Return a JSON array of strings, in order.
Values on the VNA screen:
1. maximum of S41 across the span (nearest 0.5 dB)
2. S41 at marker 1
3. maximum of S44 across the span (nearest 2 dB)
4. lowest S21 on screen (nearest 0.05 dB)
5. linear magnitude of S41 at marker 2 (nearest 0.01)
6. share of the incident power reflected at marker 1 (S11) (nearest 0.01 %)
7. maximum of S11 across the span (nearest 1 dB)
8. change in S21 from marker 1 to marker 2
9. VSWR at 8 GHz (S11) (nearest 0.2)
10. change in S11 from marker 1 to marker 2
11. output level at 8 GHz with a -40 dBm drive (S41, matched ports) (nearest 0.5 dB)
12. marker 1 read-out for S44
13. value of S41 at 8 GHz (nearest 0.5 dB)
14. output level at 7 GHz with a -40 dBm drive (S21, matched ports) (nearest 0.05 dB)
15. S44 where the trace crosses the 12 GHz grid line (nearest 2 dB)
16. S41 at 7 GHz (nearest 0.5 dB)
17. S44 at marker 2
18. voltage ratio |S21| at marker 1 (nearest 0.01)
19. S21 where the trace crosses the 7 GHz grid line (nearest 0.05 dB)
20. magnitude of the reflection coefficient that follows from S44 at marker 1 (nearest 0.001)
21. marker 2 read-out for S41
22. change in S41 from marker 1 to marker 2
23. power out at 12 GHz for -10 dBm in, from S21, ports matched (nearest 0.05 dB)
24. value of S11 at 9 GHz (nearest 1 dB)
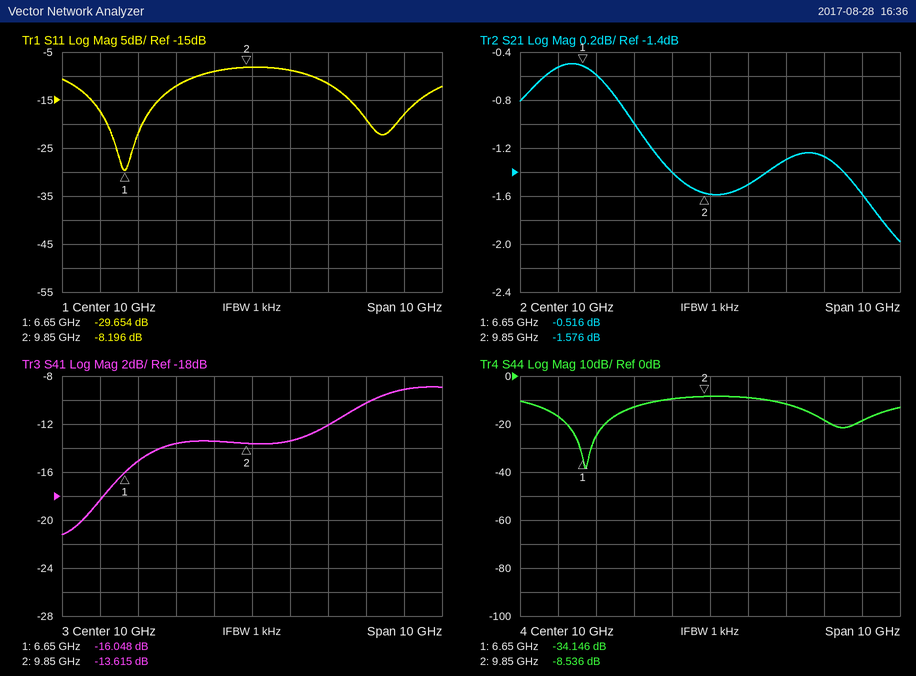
["-9.0 dB", "-16.048 dB", "-8 dB", "-2.00 dB", "0.21", "0.11 %", "-8 dB", "-1.060 dB", "1.6", "21.458 dB", "-53.5 dBm", "-34.146 dB", "-13.5 dB", "-40.60 dBm", "-12 dB", "-15.0 dB", "-8.536 dB", "0.94", "-0.60 dB", "0.020", "-13.615 dB", "2.433 dB", "-11.30 dBm", "-9 dB"]
